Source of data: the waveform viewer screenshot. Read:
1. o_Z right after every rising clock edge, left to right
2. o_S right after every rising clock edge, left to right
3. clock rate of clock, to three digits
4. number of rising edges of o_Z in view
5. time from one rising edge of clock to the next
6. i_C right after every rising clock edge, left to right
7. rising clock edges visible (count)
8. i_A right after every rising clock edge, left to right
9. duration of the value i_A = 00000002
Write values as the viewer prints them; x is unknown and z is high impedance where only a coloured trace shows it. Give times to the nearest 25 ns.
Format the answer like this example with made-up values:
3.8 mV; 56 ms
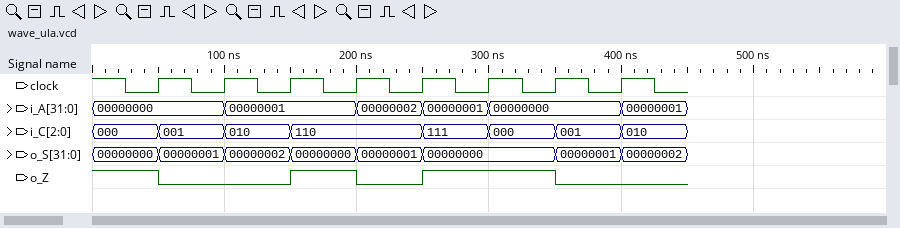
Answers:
0 0 1 0 1 1 0 0; 00000001, 00000002, 00000000, 00000001, 00000000, 00000000, 00000001, 00000002; 20.0 MHz; 2; 50 ns; 001, 010, 110, 110, 111, 000, 001, 010; 8; 00000000, 00000001, 00000001, 00000002, 00000001, 00000000, 00000000, 00000001; 50 ns
